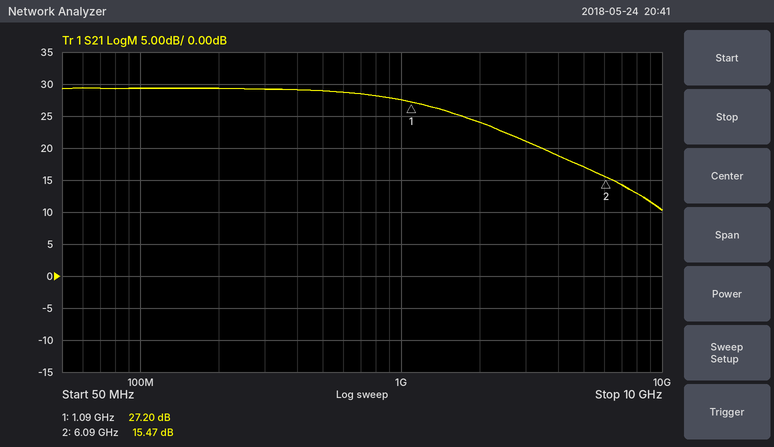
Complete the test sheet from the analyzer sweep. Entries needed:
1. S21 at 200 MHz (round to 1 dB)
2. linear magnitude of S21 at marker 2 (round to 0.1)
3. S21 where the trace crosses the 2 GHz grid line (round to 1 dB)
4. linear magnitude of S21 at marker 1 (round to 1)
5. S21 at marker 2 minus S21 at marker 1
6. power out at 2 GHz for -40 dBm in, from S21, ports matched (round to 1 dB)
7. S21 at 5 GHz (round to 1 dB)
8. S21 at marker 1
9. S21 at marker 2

29 dB
5.9
24 dB
23
-11.73 dB
-16 dBm
17 dB
27.20 dB
15.47 dB
